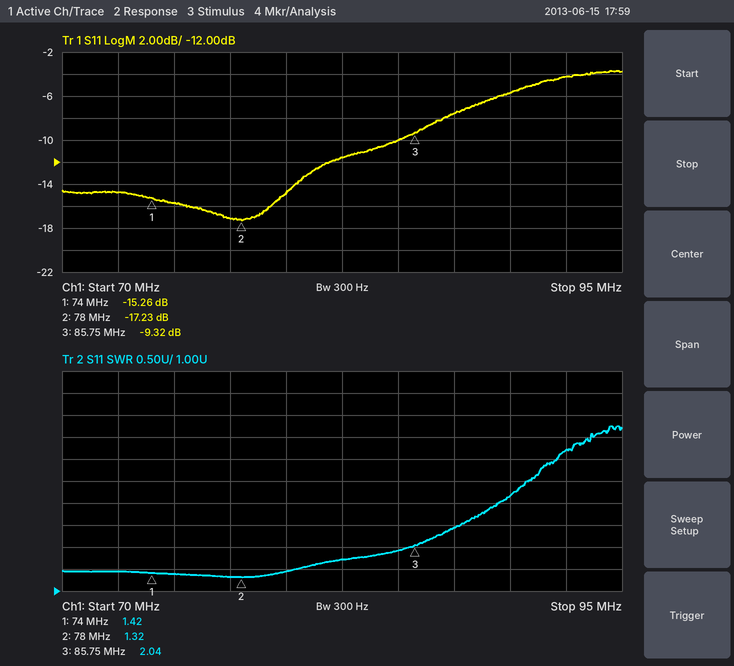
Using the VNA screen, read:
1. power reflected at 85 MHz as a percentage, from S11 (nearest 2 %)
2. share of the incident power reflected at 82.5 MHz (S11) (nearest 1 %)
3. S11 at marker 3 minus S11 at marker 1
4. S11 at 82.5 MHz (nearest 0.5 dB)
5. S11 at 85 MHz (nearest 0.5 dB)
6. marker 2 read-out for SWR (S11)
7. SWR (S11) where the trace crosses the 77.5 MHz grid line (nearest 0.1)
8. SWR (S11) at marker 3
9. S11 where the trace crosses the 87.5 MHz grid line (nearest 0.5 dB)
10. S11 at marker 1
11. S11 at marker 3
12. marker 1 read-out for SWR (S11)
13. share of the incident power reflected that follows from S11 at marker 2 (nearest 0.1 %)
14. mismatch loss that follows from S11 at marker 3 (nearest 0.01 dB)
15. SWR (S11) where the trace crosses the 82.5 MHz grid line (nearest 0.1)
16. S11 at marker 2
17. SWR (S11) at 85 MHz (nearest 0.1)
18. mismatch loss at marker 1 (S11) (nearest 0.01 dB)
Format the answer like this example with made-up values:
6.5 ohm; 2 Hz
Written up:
10 %; 7 %; 5.94 dB; -11.5 dB; -10.0 dB; 1.32; 1.3; 2.04; -7.5 dB; -15.26 dB; -9.32 dB; 1.42; 1.9 %; 0.54 dB; 1.7; -17.23 dB; 1.9; 0.13 dB
